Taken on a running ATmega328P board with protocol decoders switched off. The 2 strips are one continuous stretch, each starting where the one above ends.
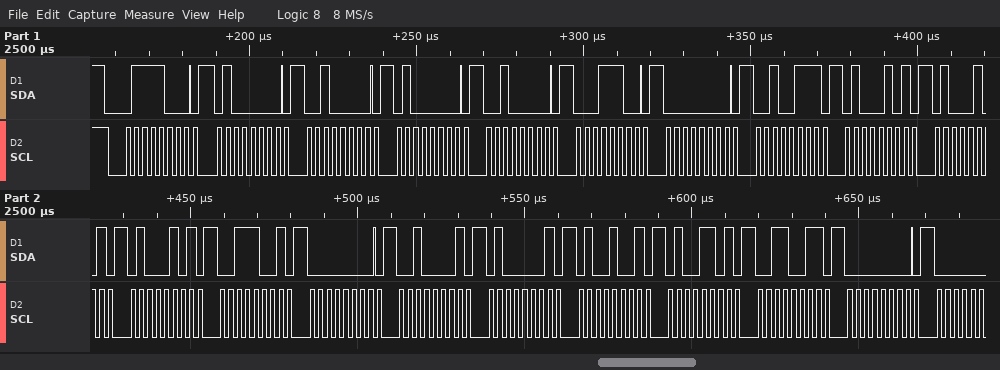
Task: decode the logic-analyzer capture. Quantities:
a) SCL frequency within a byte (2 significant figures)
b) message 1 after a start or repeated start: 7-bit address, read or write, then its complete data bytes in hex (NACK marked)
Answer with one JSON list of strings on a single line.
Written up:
["400 kHz", "0x3C write: 40 20 40 20 1C 00 27 45 45 45 39 00 21 41 49 4D 33 00"]
